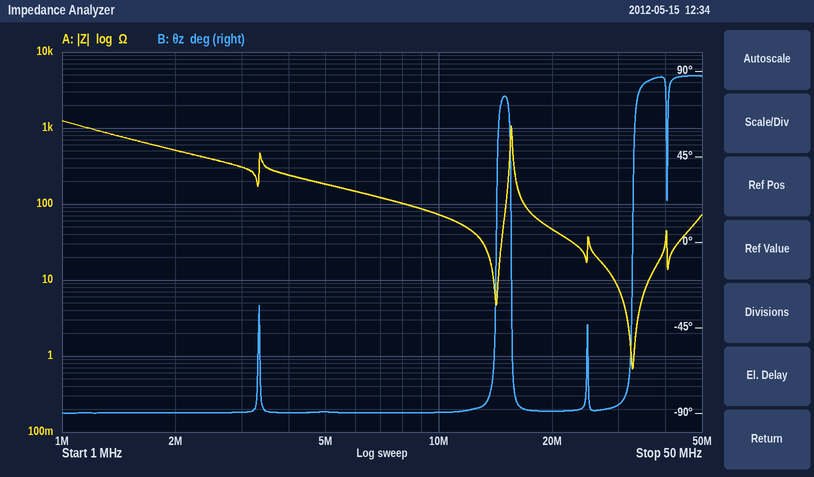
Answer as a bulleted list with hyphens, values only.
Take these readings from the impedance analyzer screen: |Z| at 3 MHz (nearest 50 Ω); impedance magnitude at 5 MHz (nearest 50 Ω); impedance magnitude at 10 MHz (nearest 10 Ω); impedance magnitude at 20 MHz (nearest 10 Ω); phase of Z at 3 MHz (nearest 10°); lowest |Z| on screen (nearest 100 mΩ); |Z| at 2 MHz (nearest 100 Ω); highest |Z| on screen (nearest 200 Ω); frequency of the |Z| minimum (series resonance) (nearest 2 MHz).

- 300 Ω
- 200 Ω
- 70 Ω
- 50 Ω
- -90°
- 700 mΩ
- 500 Ω
- 1.2 kΩ
- 32 MHz
